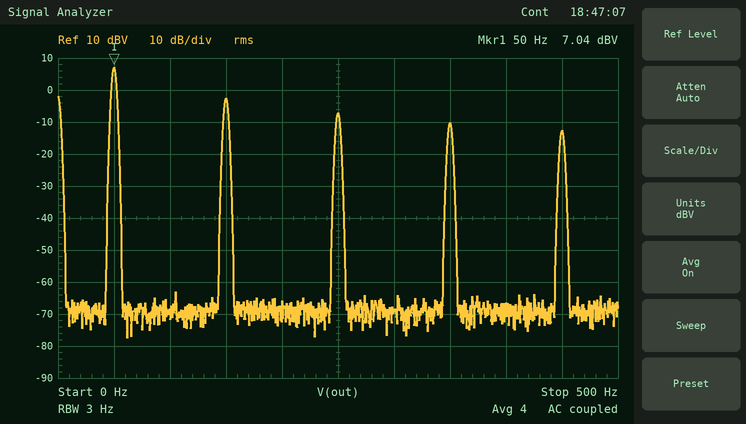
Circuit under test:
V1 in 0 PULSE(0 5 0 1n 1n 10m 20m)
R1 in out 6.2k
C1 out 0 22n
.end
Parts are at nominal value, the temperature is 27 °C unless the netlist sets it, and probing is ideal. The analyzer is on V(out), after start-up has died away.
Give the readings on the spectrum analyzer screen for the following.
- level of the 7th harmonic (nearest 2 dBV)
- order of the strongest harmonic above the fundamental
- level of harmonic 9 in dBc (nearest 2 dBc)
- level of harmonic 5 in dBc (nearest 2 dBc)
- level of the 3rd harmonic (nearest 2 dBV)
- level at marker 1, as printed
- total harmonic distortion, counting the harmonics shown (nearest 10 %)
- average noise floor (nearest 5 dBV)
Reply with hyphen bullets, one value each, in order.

- -10 dBV
- 3
- -20 dBc
- -14 dBc
- -2 dBV
- 7.04 dBV
- 40 %
- -70 dBV
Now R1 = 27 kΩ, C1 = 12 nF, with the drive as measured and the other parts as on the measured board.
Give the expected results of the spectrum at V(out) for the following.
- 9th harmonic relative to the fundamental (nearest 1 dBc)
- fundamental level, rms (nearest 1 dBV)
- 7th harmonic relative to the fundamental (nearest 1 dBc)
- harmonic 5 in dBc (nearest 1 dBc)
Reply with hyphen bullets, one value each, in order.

- -22 dBc
- 7 dBV
- -19 dBc
- -15 dBc
